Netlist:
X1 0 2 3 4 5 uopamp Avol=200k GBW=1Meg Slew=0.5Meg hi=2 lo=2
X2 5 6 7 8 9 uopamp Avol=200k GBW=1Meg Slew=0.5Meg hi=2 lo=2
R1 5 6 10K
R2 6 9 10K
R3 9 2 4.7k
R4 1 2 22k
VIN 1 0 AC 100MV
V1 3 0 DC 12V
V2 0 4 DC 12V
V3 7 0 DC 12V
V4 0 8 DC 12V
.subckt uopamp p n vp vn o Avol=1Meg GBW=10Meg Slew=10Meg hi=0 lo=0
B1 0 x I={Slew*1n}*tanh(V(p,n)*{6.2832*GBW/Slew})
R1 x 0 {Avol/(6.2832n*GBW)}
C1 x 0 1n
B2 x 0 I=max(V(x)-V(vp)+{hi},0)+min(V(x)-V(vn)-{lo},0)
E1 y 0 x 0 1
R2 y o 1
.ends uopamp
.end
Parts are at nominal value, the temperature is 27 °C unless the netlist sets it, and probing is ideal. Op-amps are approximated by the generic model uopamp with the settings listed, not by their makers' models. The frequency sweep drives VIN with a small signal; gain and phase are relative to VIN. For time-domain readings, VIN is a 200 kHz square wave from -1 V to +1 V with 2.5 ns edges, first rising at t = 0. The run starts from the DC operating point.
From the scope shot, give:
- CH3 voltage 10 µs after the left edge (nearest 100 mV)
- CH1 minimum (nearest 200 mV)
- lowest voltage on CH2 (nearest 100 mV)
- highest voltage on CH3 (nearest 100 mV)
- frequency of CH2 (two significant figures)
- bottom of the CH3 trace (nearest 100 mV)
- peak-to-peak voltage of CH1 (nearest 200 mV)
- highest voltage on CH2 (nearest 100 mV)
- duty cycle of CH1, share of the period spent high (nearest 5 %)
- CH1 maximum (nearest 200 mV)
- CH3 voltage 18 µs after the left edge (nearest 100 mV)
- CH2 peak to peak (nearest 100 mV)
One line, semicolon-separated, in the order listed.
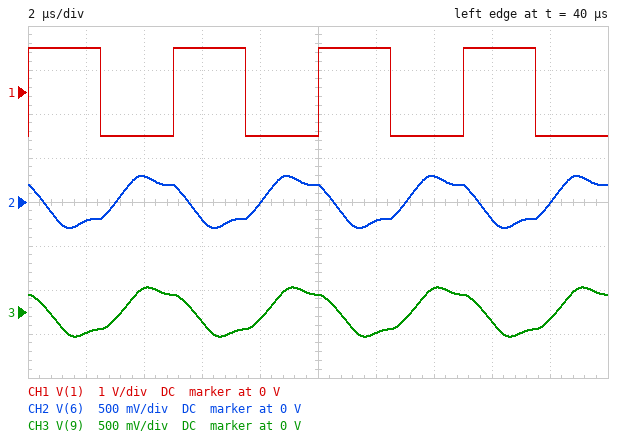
200 mV; -1.0 V; -300 mV; 300 mV; 200 kHz; -300 mV; 2.0 V; 300 mV; 50 %; 1.0 V; -100 mV; 600 mV
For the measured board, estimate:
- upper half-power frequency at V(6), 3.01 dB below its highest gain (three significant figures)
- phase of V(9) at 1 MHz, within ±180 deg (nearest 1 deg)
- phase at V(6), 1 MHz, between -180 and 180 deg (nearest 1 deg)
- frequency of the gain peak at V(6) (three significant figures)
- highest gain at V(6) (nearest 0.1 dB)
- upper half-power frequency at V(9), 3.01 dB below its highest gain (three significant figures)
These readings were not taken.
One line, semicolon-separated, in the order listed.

808 kHz; 40 deg; 85 deg; 566 kHz; -9.4 dB; 763 kHz
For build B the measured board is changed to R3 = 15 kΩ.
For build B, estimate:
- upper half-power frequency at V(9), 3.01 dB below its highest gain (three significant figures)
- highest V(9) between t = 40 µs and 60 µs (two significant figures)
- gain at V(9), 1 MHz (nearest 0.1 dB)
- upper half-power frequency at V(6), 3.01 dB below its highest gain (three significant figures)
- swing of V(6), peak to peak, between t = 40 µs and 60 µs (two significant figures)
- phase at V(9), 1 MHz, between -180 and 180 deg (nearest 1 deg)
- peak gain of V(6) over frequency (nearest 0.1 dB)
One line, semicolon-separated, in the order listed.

644 kHz; 500 mV; -12.6 dB; 683 kHz; 1.0 V; 35 deg; -0.8 dB
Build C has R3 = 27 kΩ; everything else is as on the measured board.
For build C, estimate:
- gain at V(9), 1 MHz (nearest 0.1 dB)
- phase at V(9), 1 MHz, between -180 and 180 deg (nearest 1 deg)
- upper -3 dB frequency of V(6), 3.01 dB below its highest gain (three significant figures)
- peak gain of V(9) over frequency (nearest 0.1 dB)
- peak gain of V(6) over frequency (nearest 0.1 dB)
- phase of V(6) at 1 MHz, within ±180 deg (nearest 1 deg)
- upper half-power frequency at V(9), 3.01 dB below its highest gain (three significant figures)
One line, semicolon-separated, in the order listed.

-10.5 dB; 33 deg; 582 kHz; 2.7 dB; 3.2 dB; 78 deg; 548 kHz
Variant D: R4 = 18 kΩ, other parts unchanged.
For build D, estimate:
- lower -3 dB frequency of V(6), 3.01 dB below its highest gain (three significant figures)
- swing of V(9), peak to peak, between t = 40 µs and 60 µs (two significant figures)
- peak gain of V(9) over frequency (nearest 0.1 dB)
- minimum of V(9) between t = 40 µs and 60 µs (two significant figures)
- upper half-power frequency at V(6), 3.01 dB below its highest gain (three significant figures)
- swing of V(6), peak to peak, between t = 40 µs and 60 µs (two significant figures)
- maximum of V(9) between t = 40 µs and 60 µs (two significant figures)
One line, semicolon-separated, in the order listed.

209 kHz; 670 mV; -8.9 dB; -330 mV; 793 kHz; 700 mV; 330 mV
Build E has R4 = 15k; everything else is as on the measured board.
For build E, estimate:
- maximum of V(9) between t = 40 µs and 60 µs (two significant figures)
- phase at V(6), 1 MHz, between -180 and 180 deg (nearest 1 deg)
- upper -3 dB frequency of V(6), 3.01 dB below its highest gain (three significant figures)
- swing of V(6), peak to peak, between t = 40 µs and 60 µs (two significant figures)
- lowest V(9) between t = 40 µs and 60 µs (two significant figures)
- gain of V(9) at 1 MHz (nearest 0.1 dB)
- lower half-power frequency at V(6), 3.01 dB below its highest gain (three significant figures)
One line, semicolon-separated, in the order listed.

390 mV; 84 deg; 777 kHz; 820 mV; -390 mV; -16.5 dB; 181 kHz
